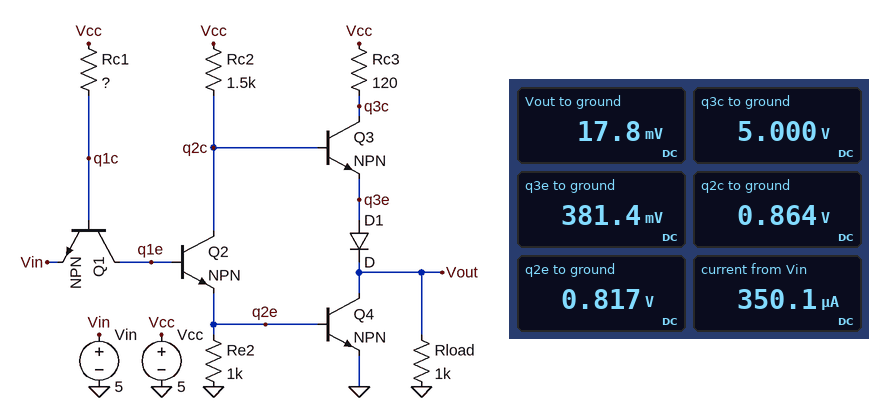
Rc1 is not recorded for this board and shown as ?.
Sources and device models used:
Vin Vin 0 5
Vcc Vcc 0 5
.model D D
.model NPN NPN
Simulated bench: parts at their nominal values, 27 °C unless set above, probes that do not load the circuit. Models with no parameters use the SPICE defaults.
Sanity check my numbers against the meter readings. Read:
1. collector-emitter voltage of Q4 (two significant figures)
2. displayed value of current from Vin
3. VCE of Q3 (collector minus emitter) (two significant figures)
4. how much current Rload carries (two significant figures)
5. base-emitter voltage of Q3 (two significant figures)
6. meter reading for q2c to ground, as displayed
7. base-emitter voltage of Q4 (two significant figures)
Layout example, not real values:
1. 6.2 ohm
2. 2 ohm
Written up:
1. 18 mV
2. 350.1 µA
3. 4.6 V
4. 18 µA
5. 480 mV
6. 0.864 V
7. 820 mV
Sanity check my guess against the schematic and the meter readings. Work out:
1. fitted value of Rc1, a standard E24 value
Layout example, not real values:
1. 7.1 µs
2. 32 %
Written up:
1. 7.5 kΩ
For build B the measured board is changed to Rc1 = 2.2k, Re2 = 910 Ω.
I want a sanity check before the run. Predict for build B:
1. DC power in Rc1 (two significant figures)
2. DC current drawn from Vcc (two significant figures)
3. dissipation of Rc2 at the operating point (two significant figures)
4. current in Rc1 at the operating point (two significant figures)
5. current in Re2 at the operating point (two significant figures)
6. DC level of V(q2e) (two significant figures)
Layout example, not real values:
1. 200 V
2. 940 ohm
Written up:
1. 3.0 mW
2. 3.9 mA
3. 11 mW
4. 1.2 mA
5. 910 µA
6. 830 mV
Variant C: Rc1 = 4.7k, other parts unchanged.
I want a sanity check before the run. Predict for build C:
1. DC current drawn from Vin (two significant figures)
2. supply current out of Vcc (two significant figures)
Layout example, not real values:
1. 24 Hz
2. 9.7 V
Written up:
1. 550 µA
2. 3.3 mA
